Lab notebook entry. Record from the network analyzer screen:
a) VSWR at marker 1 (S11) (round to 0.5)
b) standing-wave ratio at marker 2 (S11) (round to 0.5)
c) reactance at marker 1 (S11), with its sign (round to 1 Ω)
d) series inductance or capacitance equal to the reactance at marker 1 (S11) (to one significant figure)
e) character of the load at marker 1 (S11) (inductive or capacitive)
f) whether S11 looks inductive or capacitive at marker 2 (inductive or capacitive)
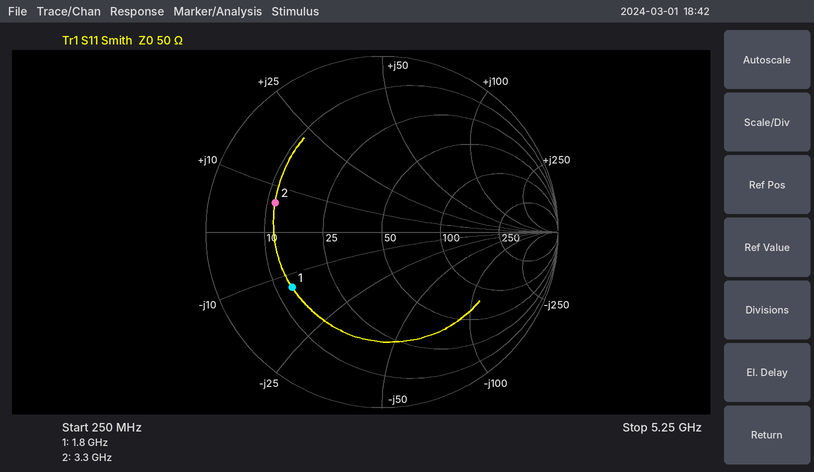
4.0
4.5
-13 Ω
7 pF
capacitive
inductive
